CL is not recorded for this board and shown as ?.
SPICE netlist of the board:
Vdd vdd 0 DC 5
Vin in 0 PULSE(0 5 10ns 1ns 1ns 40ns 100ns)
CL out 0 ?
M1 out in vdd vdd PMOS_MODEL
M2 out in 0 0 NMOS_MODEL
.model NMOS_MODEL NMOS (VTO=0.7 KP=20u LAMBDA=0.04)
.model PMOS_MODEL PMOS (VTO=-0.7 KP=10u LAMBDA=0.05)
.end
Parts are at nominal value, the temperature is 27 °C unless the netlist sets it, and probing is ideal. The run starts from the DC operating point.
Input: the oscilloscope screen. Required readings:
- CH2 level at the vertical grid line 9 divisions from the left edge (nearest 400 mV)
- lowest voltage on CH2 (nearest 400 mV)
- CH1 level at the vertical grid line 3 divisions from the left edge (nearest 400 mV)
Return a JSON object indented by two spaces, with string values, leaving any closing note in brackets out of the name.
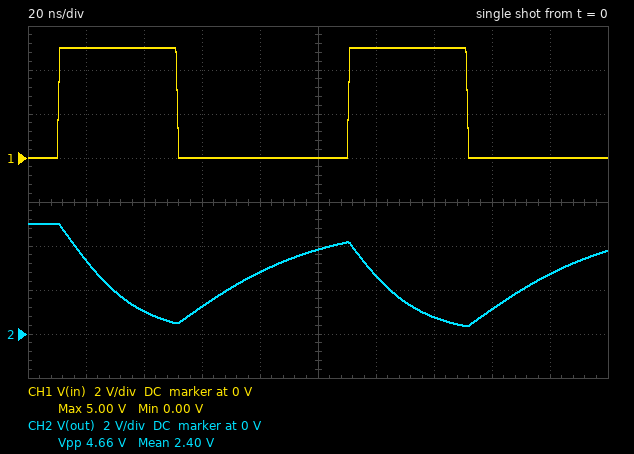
{
  "CH2 level at the vertical grid line 9 divisions from the left edge": "2.8 V",
  "lowest voltage on CH2": "400 mV",
  "CH1 level at the vertical grid line 3 divisions from the left edge": "0 V"
}
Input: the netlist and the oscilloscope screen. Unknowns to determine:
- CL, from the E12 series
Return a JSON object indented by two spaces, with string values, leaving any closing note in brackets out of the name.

{
  "CL, from the E12 series": "1.2 pF"
}
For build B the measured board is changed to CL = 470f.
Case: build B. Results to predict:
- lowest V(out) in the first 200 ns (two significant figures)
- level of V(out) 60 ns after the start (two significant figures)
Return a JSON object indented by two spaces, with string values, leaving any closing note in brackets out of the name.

{
  "lowest V(out) in the first 200 ns": "5.5 mV",
  "level of V(out) 60 ns after the start": "1.9 V"
}
